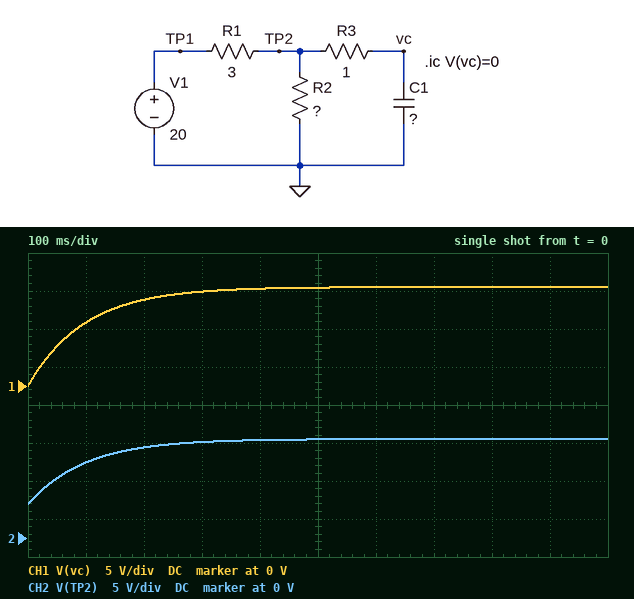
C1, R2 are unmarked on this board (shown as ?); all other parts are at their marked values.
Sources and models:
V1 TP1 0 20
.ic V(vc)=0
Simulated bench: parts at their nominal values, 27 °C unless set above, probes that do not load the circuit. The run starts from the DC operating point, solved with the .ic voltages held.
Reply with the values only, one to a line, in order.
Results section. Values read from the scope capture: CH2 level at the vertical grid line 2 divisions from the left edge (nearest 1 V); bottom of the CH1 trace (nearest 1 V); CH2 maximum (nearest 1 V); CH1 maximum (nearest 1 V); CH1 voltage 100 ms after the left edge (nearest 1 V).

12 V
0 V
13 V
13 V
8 V
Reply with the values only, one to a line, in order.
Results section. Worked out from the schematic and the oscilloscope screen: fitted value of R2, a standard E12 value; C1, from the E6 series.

5.6 Ω
33 mF
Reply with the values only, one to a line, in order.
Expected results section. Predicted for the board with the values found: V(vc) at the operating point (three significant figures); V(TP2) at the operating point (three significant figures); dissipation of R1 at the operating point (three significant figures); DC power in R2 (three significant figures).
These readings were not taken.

13.0 V
13.0 V
16.2 W
30.3 W
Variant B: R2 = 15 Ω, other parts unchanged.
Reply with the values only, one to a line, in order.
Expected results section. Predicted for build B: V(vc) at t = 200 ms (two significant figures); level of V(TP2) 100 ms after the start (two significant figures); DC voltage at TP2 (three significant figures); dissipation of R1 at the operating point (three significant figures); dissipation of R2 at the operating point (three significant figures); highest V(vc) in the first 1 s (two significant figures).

14 V
12 V
16.7 V
3.70 W
18.5 W
17 V
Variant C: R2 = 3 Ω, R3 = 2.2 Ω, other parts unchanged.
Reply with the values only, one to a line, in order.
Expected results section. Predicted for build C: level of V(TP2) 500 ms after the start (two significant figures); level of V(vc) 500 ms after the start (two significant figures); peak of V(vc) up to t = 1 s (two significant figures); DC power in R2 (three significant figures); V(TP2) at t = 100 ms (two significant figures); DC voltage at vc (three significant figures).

9.9 V
9.8 V
10 V
33.3 W
8.2 V
10.0 V
